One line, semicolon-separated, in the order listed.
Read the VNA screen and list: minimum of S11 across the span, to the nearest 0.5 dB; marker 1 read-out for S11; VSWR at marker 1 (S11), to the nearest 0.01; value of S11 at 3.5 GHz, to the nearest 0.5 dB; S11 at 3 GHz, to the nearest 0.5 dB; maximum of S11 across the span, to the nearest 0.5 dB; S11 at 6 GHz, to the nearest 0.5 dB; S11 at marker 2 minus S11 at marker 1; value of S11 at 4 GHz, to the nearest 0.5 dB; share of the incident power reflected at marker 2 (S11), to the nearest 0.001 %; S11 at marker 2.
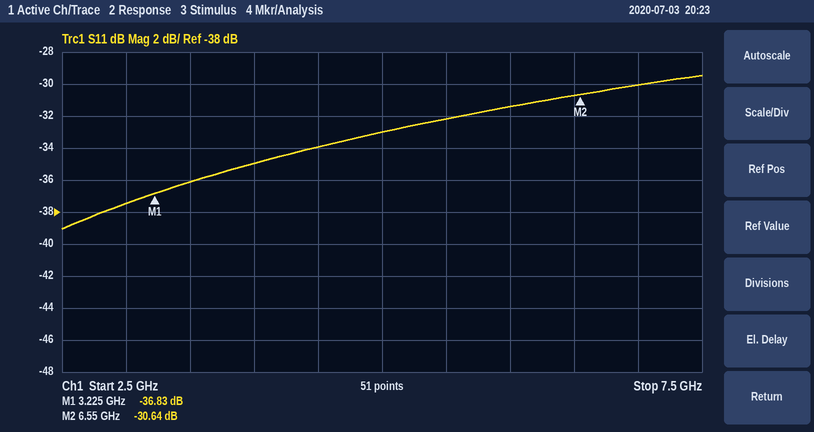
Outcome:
-39.0 dB; -36.83 dB; 1.03; -36.0 dB; -37.5 dB; -29.5 dB; -31.5 dB; 6.19 dB; -35.0 dB; 0.086 %; -30.64 dB
